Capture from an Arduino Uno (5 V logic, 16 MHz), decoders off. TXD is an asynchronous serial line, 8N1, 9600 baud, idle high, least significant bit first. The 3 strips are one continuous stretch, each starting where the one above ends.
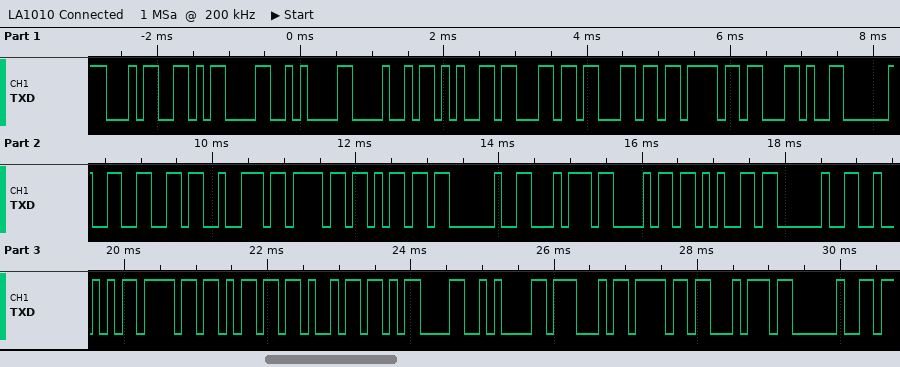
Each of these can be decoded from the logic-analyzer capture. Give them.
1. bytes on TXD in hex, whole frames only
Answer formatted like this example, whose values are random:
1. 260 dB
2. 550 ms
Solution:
1. 34 0D 0A 48 65 6C 6C 6F 2C 20 66 72 6F 6D 20 74 68 65 20 52 6F 6D 69 0D 0A 47 6F 74 20
